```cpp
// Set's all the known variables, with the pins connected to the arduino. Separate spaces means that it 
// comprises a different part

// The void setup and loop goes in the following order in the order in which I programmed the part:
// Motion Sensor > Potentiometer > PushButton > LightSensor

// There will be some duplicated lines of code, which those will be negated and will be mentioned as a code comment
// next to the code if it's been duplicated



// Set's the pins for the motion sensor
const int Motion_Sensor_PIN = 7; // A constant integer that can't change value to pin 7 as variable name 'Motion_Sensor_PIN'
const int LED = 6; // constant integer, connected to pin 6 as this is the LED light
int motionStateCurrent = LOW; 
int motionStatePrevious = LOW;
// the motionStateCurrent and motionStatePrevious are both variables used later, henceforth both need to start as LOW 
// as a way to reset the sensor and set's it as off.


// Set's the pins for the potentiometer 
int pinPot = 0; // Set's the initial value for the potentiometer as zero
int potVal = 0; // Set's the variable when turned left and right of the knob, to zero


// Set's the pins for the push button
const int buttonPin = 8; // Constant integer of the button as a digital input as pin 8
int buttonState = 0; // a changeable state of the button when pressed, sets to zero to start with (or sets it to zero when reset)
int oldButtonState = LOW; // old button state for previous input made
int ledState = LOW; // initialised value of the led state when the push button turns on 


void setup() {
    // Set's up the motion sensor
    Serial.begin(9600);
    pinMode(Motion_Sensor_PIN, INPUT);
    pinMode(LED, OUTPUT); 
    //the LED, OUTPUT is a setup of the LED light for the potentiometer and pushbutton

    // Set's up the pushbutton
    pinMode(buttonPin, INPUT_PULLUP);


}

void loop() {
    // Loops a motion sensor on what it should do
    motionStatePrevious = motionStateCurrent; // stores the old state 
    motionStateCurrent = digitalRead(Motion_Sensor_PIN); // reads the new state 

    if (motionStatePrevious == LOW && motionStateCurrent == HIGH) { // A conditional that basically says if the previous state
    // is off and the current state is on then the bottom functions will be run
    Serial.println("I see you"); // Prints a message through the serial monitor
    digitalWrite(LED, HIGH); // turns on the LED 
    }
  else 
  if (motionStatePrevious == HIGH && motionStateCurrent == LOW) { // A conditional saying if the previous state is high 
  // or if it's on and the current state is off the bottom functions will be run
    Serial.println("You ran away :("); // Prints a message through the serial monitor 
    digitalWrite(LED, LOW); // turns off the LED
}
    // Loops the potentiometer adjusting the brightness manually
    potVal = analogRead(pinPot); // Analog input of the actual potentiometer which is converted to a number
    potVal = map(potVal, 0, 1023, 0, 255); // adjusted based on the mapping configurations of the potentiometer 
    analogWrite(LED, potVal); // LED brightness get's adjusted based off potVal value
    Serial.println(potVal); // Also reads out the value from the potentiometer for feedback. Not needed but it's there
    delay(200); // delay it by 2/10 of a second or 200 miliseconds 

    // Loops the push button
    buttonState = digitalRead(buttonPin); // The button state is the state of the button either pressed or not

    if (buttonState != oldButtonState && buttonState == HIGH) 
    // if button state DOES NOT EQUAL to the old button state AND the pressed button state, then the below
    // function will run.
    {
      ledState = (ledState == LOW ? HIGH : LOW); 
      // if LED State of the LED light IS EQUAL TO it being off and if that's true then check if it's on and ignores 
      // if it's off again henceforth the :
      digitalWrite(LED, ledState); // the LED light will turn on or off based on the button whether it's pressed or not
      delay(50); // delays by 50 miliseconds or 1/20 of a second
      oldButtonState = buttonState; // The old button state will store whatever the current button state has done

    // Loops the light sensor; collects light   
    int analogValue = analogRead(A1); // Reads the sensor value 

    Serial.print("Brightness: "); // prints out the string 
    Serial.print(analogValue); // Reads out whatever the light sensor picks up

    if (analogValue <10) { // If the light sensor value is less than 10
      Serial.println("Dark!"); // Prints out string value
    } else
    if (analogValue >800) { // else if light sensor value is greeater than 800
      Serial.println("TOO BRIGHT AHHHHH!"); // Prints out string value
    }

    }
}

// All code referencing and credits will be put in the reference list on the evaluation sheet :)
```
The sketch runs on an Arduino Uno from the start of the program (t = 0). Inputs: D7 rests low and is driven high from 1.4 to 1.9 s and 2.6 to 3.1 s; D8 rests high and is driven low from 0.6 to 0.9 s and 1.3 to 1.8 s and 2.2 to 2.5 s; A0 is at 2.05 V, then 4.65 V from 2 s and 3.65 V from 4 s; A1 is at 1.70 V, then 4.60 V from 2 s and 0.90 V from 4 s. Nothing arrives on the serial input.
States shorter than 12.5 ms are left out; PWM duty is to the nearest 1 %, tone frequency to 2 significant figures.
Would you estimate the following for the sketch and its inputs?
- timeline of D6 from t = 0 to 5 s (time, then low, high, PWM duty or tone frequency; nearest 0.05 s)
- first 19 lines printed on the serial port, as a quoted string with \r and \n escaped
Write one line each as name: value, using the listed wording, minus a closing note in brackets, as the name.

timeline of D6 from t = 0 to 5 s: 0 s PWM 41 %; 0.2 s high; 0.25 s PWM 41 %; 2.05 s PWM 93 %; 4.05 s PWM 73 %
first 19 lines printed on the serial port, as a quoted string with \r and \n escaped: "104\r\nBrightness: 348104\r\n104\r\n104\r\n104\r\n104\r\n104\r\nI see you\r\n104\r\n104\r\n104\r\nYou ran away :(\r\n237\r\n237\r\n237\r\nI see you\r\n237\r\n237\r\n237\r\n"
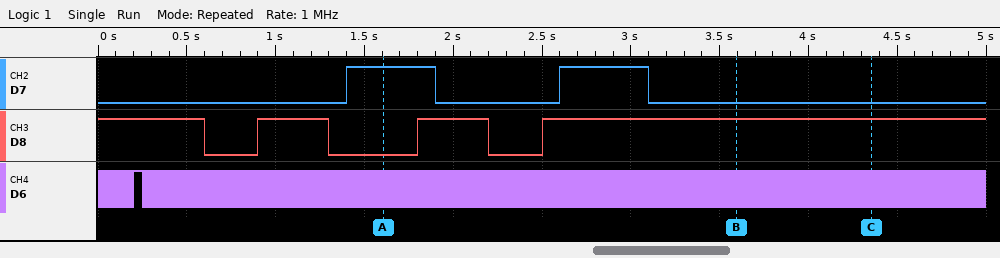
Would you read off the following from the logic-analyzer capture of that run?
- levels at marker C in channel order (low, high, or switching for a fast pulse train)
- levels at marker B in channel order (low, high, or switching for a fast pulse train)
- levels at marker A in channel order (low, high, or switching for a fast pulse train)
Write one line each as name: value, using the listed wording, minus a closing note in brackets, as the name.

levels at marker C in channel order: D7 low, D8 high, D6 switching
levels at marker B in channel order: D7 low, D8 high, D6 switching
levels at marker A in channel order: D7 high, D8 low, D6 switching
